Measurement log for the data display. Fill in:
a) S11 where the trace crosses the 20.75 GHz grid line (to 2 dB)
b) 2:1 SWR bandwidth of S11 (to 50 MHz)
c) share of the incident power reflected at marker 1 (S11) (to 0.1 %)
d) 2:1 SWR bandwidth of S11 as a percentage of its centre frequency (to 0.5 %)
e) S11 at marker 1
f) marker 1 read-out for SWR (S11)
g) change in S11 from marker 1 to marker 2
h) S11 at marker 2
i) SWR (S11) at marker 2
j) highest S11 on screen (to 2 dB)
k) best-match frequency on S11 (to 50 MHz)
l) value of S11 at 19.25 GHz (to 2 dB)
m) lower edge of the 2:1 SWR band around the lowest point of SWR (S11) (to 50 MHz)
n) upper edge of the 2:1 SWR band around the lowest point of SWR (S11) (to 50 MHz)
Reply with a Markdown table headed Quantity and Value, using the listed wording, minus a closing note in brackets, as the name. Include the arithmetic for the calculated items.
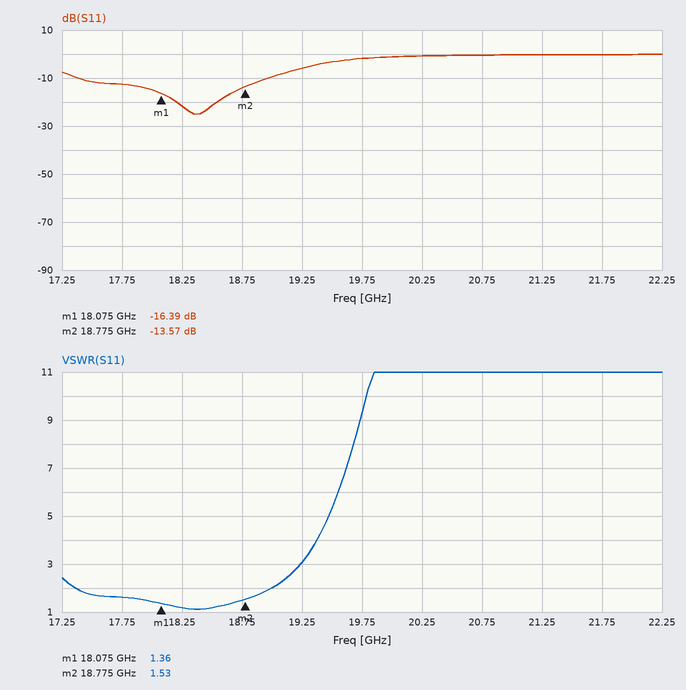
| Quantity | Value |
|---|---|
| S11 where the trace crosses the 20.75 GHz grid line | 0 dB |
| 2:1 SWR bandwidth of S11 | 19.00 GHz − 17.35 GHz = 1.65 GHz |
| share of the incident power reflected at marker 1 (S11) | 10^(-16.39/10) ≈ 2.3 % |
| 2:1 SWR bandwidth of S11 as a percentage of its centre frequency | 1.65 GHz / 18.175 GHz ≈ 9.08 %, so 9.0 % to the nearest 0.5 % |
| S11 at marker 1 | -16.39 dB |
| marker 1 read-out for SWR | 1.36 |
| change in S11 from marker 1 to marker 2 | -13.57 − (-16.39) = 2.82 dB |
| S11 at marker 2 | -13.57 dB |
| SWR (S11) at marker 2 | 1.53 |
| highest S11 on screen | 0 dB |
| best-match frequency on S11 | 18.35 GHz |
| value of S11 at 19.25 GHz | -6 dB |
| lower edge of the 2:1 SWR band around the lowest point of SWR (S11) | 17.35 GHz |
| upper edge of the 2:1 SWR band around the lowest point of SWR (S11) | 19.00 GHz |
